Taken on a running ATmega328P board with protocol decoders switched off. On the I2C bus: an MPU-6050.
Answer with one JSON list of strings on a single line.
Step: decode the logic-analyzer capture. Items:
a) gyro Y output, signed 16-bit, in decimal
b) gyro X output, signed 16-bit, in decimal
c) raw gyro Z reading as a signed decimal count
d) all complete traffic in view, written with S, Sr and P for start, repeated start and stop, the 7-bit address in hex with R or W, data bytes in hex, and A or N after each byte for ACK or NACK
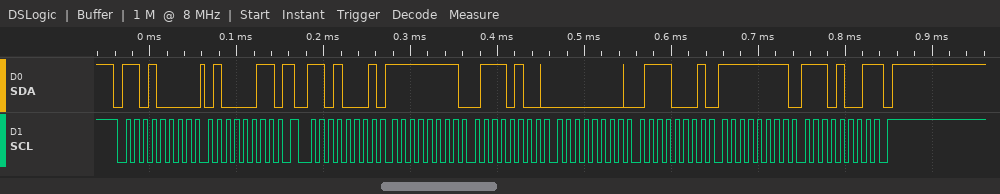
["113", "-140", "-23", "S 68W A 43 A Sr 68R A FF A 74 A 00 A 71 A FF A E9 N P"]
